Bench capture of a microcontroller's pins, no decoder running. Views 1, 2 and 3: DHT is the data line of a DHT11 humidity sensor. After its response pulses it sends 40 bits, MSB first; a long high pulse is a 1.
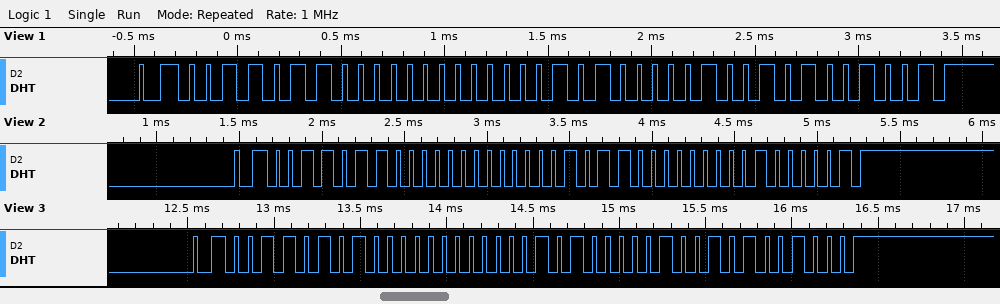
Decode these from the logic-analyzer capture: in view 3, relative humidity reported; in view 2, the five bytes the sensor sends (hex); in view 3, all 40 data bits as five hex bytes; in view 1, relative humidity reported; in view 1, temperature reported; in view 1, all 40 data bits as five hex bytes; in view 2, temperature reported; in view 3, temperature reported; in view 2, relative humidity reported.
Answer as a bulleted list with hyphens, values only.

- 53 %
- 36 00 0B 00 41
- 35 00 0A 09 48
- 54 %
- 10.9 °C
- 36 00 0A 09 49
- 11.0 °C
- 10.9 °C
- 54 %
